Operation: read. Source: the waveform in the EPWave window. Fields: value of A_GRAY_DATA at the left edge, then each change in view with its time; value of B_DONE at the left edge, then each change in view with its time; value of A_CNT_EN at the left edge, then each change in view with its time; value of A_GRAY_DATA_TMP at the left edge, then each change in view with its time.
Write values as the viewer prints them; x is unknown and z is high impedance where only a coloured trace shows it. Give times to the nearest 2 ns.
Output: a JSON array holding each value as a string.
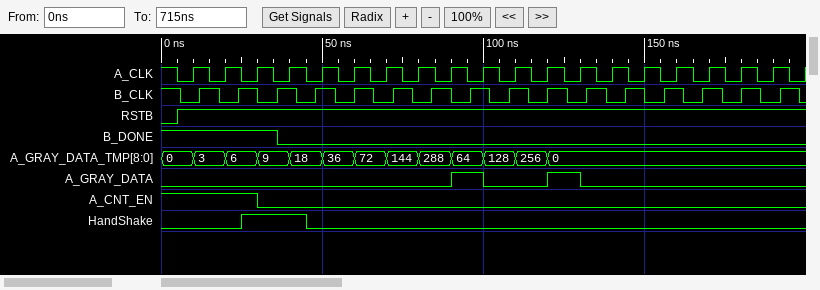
["0, 1 at 90 ns, 0 at 100 ns, 1 at 120 ns, 0 at 130 ns", "1, 0 at 36 ns", "1, 0 at 30 ns", "0, 3 at 10 ns, 6 at 20 ns, 9 at 30 ns, 18 at 40 ns, 36 at 50 ns, 72 at 60 ns, 144 at 70 ns, 288 at 80 ns, 64 at 90 ns, 128 at 100 ns, 256 at 110 ns, 0 at 120 ns"]
